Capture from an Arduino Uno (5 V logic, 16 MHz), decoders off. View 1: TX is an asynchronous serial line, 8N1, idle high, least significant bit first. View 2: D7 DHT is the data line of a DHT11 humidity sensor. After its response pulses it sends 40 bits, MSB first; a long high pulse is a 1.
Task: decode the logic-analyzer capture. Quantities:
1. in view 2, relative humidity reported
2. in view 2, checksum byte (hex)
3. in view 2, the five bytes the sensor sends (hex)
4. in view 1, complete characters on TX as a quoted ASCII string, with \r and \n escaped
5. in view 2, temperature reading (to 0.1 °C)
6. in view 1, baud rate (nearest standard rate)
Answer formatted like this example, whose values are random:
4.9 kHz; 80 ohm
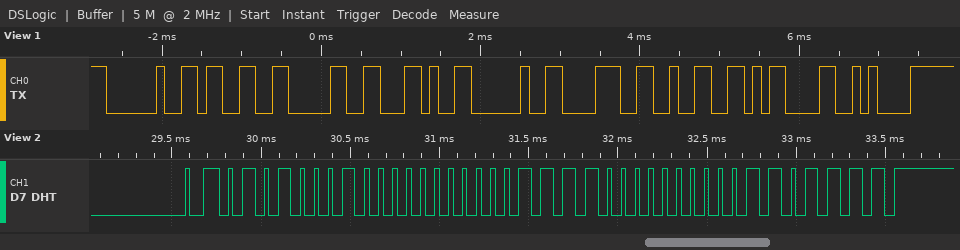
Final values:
81 %; 0x6F; 51 00 1E 00 6F; " 30, 82\r\n"; 30.0 °C; 9600 baud
